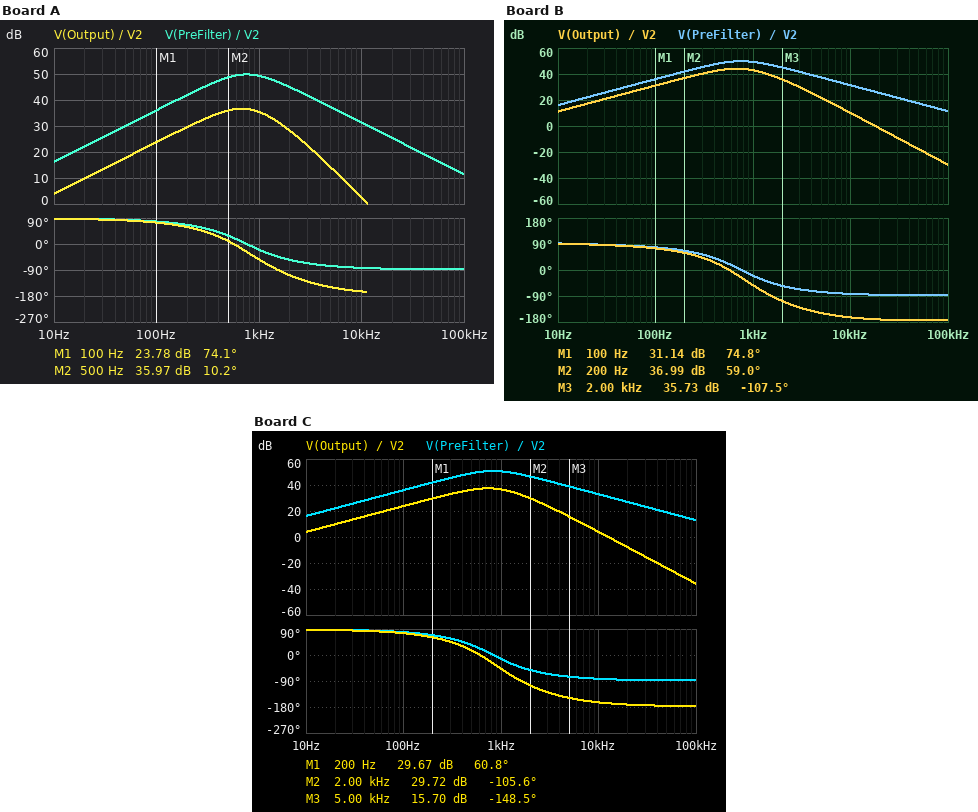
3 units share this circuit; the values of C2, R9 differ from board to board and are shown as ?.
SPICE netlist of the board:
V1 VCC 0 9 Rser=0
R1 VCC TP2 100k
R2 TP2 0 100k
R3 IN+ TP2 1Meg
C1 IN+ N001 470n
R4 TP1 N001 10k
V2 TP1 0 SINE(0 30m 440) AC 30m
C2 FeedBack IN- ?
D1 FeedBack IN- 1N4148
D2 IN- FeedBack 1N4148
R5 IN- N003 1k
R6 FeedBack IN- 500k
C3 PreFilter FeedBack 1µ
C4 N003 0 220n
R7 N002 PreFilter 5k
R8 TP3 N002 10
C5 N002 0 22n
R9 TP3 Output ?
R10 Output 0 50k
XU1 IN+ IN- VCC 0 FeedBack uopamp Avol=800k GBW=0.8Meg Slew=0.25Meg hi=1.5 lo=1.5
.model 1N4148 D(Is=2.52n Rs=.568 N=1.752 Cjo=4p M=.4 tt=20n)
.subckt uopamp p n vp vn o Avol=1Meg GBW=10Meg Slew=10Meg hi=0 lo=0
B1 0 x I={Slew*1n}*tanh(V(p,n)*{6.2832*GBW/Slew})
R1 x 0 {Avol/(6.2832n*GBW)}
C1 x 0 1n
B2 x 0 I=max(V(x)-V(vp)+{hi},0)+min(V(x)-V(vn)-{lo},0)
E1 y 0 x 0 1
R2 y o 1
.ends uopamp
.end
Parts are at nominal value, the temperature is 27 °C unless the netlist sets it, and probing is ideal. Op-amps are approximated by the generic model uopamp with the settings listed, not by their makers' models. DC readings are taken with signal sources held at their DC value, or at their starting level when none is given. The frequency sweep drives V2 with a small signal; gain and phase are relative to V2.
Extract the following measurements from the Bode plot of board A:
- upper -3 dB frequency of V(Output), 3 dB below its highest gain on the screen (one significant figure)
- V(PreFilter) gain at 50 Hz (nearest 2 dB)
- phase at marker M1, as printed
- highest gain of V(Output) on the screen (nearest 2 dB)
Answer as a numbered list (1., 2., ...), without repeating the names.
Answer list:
1. 1 kHz
2. 30 dB
3. 74.1 deg
4. 36 dB
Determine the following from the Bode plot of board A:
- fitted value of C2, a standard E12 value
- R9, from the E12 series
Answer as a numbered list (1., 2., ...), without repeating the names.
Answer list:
1. 220 pF
2. 150 kΩ
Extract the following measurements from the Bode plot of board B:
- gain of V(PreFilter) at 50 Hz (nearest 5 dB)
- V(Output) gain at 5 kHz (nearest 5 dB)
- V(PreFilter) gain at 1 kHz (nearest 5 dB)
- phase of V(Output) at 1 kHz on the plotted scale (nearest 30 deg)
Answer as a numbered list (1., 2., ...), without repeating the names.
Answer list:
1. 30 dB
2. 20 dB
3. 50 dB
4. -60 deg
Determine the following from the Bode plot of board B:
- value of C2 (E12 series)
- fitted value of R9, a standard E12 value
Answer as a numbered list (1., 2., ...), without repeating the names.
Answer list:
1. 220 pF
2. 33 kΩ
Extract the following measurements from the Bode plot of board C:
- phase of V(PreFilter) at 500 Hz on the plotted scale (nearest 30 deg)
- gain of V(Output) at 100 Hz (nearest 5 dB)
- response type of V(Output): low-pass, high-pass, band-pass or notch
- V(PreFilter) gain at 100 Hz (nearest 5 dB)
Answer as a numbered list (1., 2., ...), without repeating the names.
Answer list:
1. 30 deg
2. 25 dB
3. band-pass
4. 35 dB
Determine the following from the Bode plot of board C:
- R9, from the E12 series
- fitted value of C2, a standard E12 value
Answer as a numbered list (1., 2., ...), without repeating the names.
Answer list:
1. 150 kΩ
2. 150 pF
